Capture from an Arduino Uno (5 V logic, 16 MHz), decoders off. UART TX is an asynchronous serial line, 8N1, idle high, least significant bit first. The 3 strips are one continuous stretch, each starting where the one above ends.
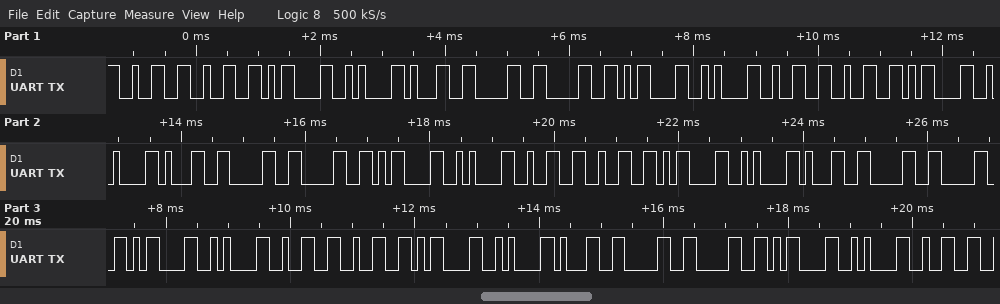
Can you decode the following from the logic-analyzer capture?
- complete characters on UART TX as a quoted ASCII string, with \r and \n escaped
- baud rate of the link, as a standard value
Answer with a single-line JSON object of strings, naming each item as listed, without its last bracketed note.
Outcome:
{"complete characters on UART TX as a quoted ASCII string, with \\r and \\n escaped": "\"22\\r\\n100\\r\\n22\\r\\n100\\r\\n22\\r\\n100\\r\\n22\\r\\n100\\r\\n2\"", "baud rate of the link, as a standard value": "9600 baud"}
